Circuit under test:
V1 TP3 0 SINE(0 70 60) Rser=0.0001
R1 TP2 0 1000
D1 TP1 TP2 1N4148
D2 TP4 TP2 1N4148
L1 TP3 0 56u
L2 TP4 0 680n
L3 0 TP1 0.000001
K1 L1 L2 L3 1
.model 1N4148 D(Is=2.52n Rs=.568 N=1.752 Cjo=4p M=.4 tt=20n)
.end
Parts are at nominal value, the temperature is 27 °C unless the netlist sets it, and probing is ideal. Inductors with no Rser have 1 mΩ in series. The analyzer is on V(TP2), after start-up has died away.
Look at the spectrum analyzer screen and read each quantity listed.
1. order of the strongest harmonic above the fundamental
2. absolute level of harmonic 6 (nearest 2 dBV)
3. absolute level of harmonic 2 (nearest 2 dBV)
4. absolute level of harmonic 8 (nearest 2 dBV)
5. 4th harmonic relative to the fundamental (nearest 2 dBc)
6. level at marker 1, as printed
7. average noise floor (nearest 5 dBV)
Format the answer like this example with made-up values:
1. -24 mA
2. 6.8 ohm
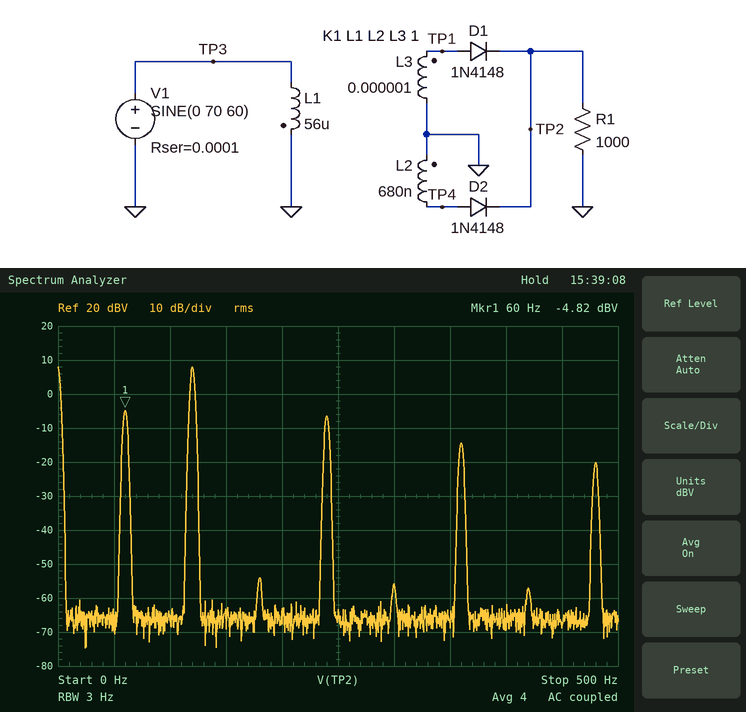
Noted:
1. 2
2. -14 dBV
3. 8 dBV
4. -20 dBV
5. -2 dBc
6. -4.82 dBV
7. -65 dBV
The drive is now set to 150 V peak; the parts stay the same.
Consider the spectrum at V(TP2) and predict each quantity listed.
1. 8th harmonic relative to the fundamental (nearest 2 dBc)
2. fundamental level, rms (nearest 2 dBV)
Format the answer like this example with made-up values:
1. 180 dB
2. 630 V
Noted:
1. -14 dBc
2. 2 dBV
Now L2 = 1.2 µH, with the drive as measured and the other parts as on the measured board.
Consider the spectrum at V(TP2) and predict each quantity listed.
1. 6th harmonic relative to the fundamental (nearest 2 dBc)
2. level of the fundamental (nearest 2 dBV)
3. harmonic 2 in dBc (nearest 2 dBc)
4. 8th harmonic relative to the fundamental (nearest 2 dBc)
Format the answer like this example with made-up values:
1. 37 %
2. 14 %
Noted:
1. -2 dBc
2. -10 dBV
3. 20 dBc
4. -8 dBc
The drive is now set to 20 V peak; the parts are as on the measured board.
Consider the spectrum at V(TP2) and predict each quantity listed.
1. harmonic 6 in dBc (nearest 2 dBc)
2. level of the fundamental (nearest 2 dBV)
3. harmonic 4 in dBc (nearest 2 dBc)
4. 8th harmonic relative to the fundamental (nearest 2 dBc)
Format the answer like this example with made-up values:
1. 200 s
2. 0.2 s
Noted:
1. -20 dBc
2. -16 dBV
3. -6 dBc
4. -40 dBc
